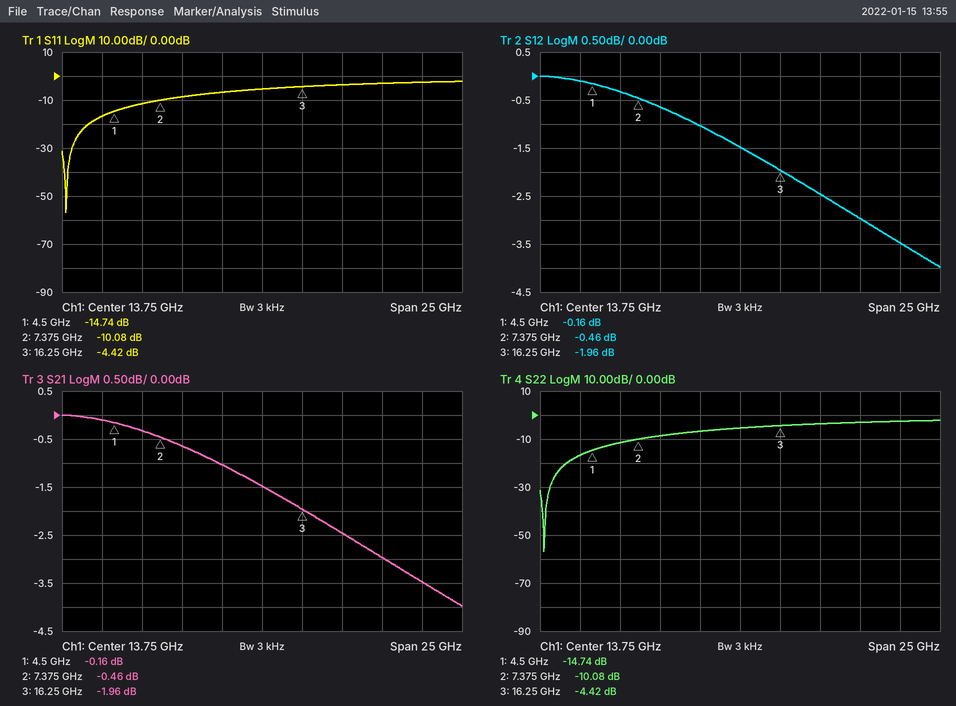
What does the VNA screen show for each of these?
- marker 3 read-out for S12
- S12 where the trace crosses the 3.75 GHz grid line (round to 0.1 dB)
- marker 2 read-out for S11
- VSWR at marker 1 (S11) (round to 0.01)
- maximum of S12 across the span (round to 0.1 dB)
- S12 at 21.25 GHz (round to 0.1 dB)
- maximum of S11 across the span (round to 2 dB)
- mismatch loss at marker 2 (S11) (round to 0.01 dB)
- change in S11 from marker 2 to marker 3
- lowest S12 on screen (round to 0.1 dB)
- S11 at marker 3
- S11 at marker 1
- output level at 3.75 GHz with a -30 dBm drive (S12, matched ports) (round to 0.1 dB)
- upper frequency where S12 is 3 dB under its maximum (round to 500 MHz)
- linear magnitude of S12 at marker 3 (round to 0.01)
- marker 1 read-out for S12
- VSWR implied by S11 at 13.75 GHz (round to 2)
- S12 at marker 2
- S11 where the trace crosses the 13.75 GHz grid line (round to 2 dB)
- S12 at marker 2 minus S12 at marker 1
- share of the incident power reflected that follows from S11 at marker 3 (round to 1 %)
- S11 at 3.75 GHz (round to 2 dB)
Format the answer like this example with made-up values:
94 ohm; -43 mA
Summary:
-1.96 dB; -0.1 dB; -10.08 dB; 1.45; 0.0 dB; -3.0 dB; -2 dB; 0.45 dB; 5.66 dB; -4.0 dB; -4.42 dB; -14.74 dB; -30.1 dBm; 21.5 GHz; 0.80; -0.16 dB; 4; -0.46 dB; -6 dB; -0.30 dB; 36 %; -16 dB
